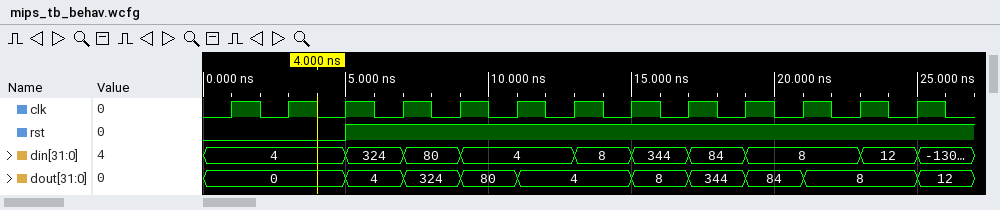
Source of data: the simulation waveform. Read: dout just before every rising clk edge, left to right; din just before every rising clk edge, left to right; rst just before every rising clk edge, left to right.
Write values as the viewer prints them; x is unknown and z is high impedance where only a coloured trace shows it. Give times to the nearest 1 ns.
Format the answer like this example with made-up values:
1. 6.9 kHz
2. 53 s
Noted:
1. 0, 0, 0, 4, 324, 80, 4, 4, 8, 344, 84, 8, 8
2. 4, 4, 4, 324, 80, 4, 4, 8, 344, 84, 8, 8, 12
3. 0 0 0 1 1 1 1 1 1 1 1 1 1
